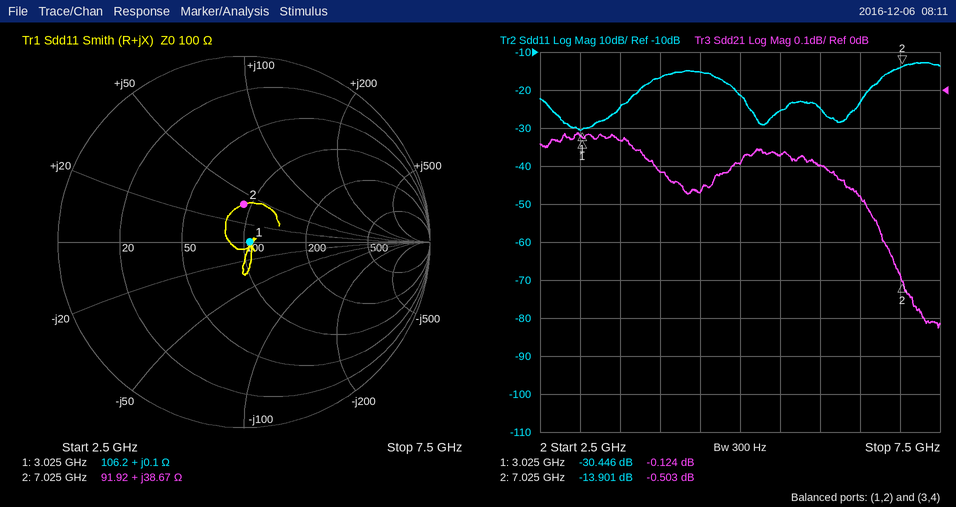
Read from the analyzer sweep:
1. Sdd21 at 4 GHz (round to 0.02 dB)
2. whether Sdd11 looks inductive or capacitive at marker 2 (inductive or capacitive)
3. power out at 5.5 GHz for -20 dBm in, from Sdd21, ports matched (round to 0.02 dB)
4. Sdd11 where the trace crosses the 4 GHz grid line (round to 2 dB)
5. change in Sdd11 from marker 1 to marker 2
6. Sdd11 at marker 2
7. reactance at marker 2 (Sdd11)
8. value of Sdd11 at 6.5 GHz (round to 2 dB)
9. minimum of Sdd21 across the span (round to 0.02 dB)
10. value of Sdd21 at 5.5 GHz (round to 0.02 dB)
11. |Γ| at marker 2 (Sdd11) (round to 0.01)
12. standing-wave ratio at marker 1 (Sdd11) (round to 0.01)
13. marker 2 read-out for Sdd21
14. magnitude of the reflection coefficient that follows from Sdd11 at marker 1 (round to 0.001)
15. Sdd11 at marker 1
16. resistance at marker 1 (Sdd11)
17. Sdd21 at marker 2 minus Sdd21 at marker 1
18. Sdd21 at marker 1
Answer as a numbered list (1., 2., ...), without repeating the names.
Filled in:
1. -0.22 dB
2. inductive
3. -20.18 dBm
4. -16 dB
5. 16.545 dB
6. -13.901 dB
7. +38.67 Ω
8. -24 dB
9. -0.62 dB
10. -0.18 dB
11. 0.20
12. 1.06
13. -0.503 dB
14. 0.030
15. -30.446 dB
16. 106.2 Ω
17. -0.379 dB
18. -0.124 dB
